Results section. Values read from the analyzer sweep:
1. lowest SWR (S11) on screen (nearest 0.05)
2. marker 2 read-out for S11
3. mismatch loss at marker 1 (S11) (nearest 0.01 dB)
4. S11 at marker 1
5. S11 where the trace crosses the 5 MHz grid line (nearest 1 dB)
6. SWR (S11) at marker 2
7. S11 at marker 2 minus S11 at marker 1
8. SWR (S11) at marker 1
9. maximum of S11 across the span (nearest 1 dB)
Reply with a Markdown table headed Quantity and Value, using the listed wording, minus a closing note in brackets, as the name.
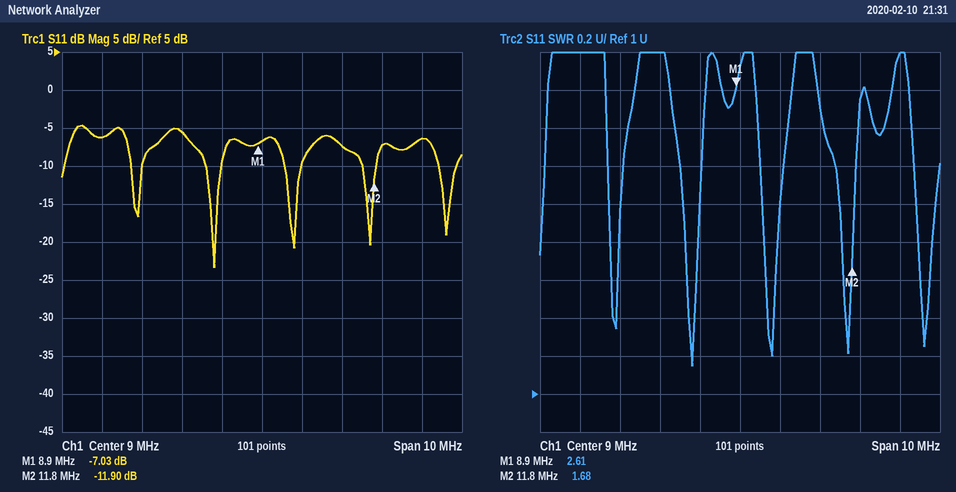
| Quantity | Value |
|---|---|
| lowest SWR (S11) on screen | 1.15 |
| marker 2 read-out for S11 | -11.90 dB |
| mismatch loss at marker 1 (S11) | 0.96 dB |
| S11 at marker 1 | -7.03 dB |
| S11 where the trace crosses the 5 MHz grid line | -6 dB |
| SWR (S11) at marker 2 | 1.68 |
| S11 at marker 2 minus S11 at marker 1 | -4.87 dB |
| SWR (S11) at marker 1 | 2.61 |
| maximum of S11 across the span | -5 dB |
